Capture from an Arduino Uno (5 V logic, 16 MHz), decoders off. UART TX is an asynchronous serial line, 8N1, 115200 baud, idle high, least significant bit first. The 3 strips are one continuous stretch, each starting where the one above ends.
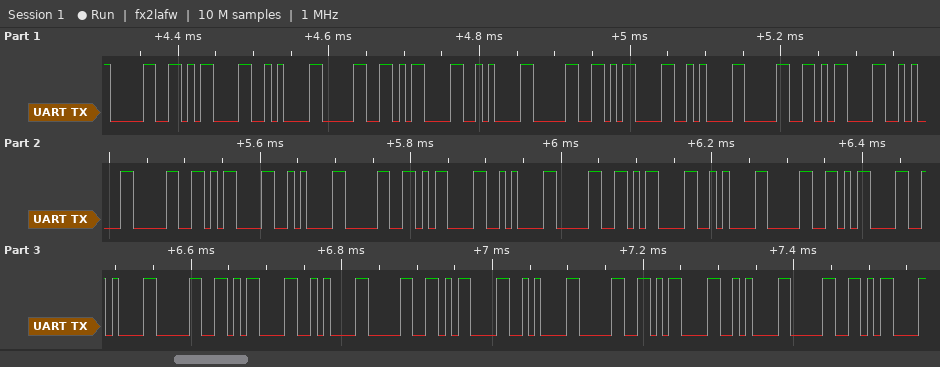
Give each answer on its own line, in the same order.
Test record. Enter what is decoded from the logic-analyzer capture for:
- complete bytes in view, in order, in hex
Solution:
30 0D 0A 30 0D 0A 30 0D 0A 30 0D 0A 30 0D 0A 30 0D 0A 30 0D 0A 30 0D 0A 30 0D 0A 30 0D 0A 30 0D 0A 30 0D
